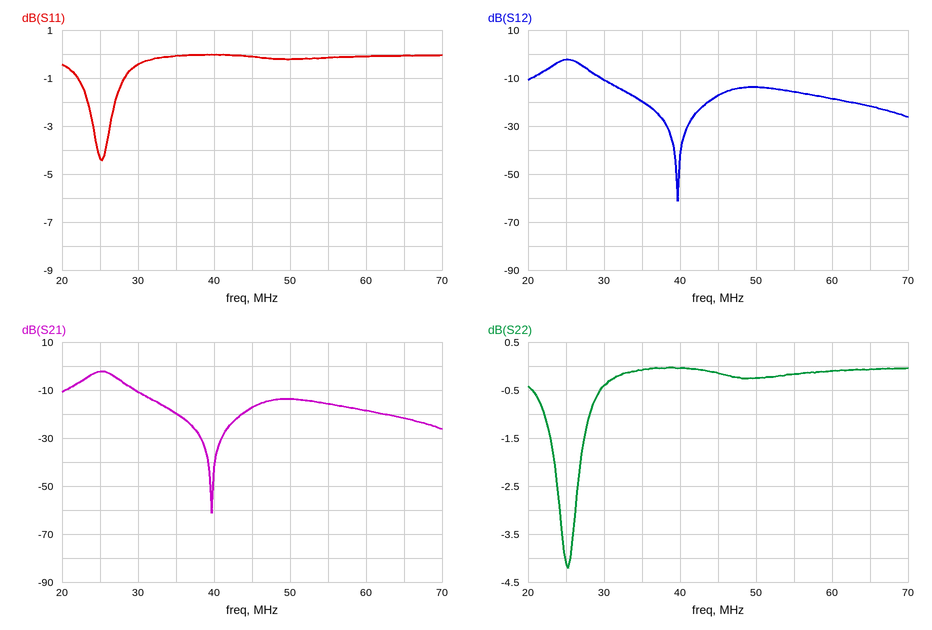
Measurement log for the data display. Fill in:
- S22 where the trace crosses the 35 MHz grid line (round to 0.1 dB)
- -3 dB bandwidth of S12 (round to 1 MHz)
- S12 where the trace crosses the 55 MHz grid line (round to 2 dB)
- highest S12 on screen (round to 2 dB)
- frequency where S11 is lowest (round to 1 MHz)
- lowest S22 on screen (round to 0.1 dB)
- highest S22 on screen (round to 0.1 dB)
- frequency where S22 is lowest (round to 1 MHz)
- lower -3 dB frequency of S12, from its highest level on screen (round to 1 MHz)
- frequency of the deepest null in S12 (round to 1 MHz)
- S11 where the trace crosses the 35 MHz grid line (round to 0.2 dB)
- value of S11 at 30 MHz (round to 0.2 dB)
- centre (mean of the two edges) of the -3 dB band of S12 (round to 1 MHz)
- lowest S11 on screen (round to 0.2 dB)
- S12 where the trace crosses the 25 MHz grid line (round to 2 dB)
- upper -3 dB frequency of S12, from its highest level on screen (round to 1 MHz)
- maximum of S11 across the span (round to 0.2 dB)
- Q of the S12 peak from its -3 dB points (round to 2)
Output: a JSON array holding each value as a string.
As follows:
["-0.1 dB", "4 MHz", "-16 dB", "-2 dB", "25 MHz", "-4.2 dB", "0.0 dB", "25 MHz", "23 MHz", "40 MHz", "0.0 dB", "-0.4 dB", "25 MHz", "-4.4 dB", "-2 dB", "27 MHz", "0.0 dB", "6"]
